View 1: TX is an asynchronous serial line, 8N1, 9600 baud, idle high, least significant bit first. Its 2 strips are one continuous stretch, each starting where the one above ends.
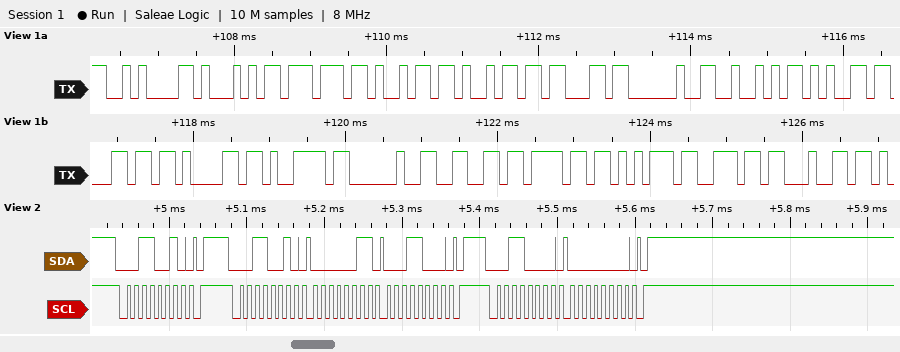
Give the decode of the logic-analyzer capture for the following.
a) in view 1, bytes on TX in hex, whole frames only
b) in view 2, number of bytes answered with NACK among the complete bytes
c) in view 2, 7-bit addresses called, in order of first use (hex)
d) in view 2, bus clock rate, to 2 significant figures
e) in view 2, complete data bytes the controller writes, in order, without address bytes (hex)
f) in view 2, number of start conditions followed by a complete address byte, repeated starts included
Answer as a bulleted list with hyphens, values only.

- 0x0A 0x51 0x77 0x69 0x69 0x63 0x20 0x52 0x65 0x6C 0x61 0x79 0x20 0x66 0x6F 0x75 0x6E 0x64
- 0
- 0x19 0x18
- 100 kHz
- 03 18 00
- 3
